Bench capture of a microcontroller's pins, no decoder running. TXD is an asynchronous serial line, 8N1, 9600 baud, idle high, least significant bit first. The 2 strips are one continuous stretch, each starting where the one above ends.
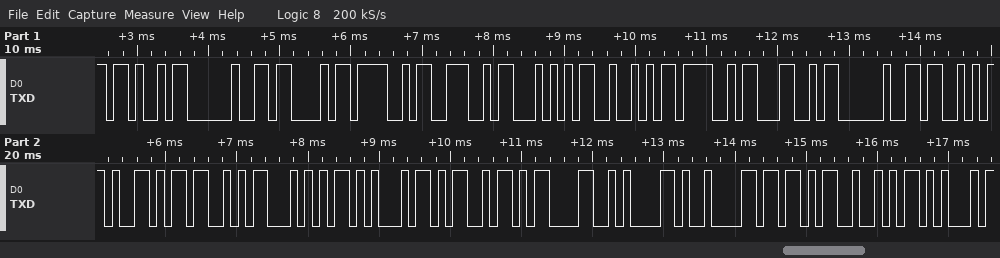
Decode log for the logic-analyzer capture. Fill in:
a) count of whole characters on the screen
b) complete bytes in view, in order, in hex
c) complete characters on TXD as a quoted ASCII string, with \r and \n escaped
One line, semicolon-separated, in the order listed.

22; 4B 20 43 4F 4E 54 52 4F 4C 20 53 59 53 54 45 4D 0D 0A 09 5B 52 45; "K CONTROL SYSTEM\r\n\t[RE"
